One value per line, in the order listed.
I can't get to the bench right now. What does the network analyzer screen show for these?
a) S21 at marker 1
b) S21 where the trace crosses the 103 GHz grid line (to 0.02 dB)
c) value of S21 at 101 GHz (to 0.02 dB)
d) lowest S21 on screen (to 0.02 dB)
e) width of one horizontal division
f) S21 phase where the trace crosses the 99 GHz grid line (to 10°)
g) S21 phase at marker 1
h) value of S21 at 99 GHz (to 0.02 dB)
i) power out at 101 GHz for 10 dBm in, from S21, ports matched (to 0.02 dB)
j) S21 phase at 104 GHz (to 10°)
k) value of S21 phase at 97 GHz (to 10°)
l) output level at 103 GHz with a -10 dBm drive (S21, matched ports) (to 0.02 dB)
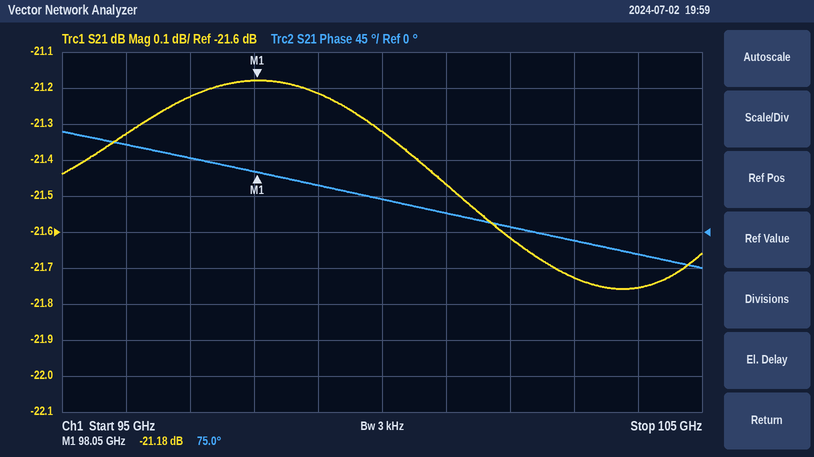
-21.18 dB
-21.72 dB
-21.46 dB
-21.76 dB
1 GHz
60°
75.0°
-21.22 dB
-11.46 dBm
-30°
90°
-31.72 dBm
